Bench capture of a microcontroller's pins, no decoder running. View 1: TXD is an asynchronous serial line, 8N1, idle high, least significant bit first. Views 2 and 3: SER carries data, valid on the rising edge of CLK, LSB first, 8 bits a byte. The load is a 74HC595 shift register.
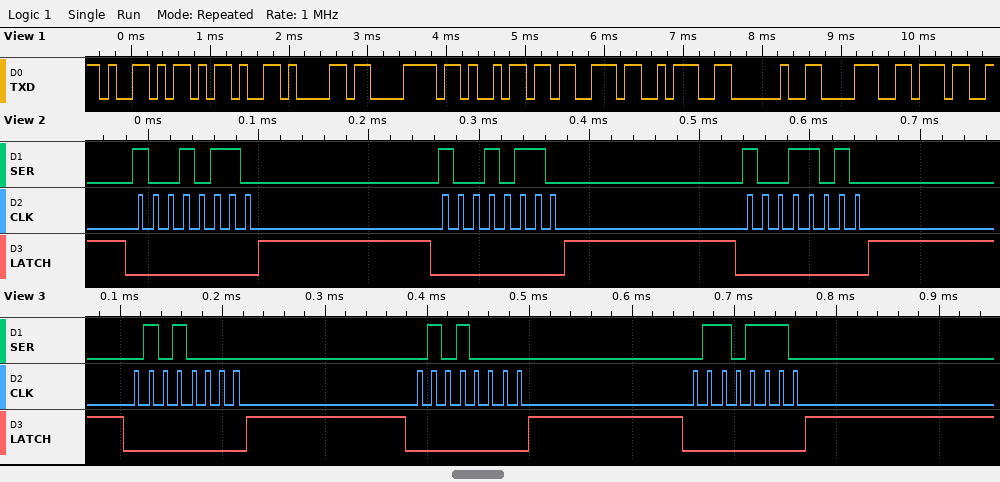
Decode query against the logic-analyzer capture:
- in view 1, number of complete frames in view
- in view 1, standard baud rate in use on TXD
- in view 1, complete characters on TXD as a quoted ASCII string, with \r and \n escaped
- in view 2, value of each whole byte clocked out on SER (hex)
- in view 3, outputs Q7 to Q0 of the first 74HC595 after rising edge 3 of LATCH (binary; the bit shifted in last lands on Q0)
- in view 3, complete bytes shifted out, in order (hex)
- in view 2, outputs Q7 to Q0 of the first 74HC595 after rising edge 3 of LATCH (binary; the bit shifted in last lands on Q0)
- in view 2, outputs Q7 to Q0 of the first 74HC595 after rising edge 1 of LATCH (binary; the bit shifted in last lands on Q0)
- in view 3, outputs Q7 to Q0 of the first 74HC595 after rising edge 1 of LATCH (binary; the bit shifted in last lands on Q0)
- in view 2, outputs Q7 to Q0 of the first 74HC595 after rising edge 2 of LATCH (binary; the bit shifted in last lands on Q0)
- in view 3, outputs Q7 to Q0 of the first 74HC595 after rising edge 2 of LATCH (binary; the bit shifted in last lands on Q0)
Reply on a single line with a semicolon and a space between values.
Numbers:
10; 9600 baud; "Y-axis: 87"; 69 69 59; 01101110; 0A 0A 76; 10011010; 10010110; 01010000; 10010110; 01010000
